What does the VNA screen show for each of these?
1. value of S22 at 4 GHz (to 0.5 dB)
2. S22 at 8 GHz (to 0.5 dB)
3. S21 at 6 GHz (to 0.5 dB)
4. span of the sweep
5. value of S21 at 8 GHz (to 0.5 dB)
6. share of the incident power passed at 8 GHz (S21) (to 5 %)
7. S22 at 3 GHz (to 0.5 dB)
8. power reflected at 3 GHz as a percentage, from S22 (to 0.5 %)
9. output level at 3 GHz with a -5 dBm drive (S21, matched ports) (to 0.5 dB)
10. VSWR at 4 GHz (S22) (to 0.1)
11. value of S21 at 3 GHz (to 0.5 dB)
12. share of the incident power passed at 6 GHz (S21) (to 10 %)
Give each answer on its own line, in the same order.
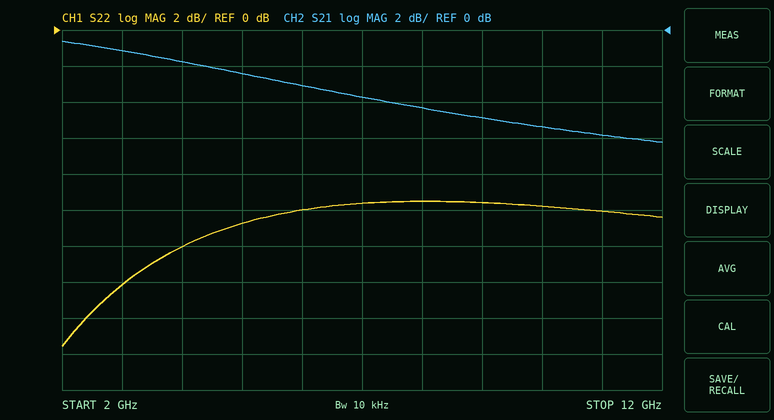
-12.0 dB
-9.5 dB
-3.0 dB
10 GHz
-4.5 dB
35 %
-14.0 dB
4.0 %
-6.0 dBm
1.7
-1.0 dB
50 %
